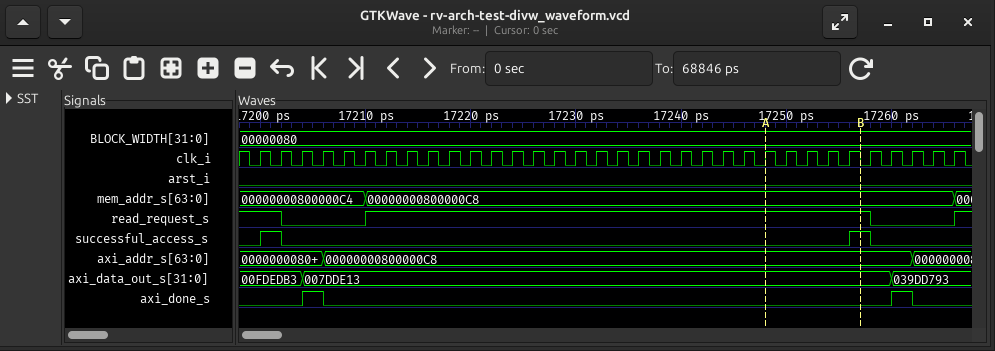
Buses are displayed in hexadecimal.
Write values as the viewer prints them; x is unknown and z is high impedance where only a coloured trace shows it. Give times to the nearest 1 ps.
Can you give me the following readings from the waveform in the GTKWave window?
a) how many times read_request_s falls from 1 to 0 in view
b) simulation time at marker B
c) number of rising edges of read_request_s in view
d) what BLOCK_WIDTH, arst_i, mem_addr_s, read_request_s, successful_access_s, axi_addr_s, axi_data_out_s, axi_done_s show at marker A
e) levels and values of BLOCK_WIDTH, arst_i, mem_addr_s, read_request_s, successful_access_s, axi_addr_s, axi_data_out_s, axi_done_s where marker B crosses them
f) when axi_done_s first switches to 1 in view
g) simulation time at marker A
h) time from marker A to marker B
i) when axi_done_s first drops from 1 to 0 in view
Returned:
2
17257 ps
2
BLOCK_WIDTH=00000080, arst_i=0, mem_addr_s=00000000800000C8, read_request_s=1, successful_access_s=0, axi_addr_s=00000000800000C8, axi_data_out_s=007DDE13, axi_done_s=0
BLOCK_WIDTH=00000080, arst_i=0, mem_addr_s=00000000800000C8, read_request_s=1, successful_access_s=1, axi_addr_s=00000000800000C8, axi_data_out_s=007DDE13, axi_done_s=0
17204 ps
17248 ps
9 ps
17206 ps
